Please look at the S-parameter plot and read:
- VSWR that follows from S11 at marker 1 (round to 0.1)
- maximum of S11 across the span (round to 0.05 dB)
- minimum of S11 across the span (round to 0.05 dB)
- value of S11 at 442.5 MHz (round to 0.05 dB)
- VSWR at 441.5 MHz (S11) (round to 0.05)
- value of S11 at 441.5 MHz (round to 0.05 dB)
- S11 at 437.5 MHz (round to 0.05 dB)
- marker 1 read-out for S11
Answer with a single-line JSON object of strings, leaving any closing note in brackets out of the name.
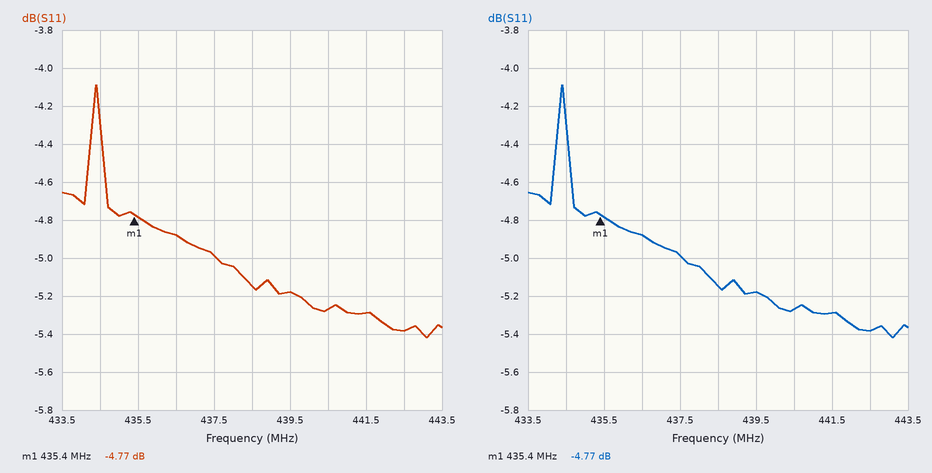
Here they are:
{"VSWR that follows from S11 at marker 1": "3.7", "maximum of S11 across the span": "-4.10 dB", "minimum of S11 across the span": "-5.40 dB", "value of S11 at 442.5 MHz": "-5.40 dB", "VSWR at 441.5 MHz (S11)": "3.40", "value of S11 at 441.5 MHz": "-5.30 dB", "S11 at 437.5 MHz": "-5.00 dB", "marker 1 read-out for S11": "-4.77 dB"}
